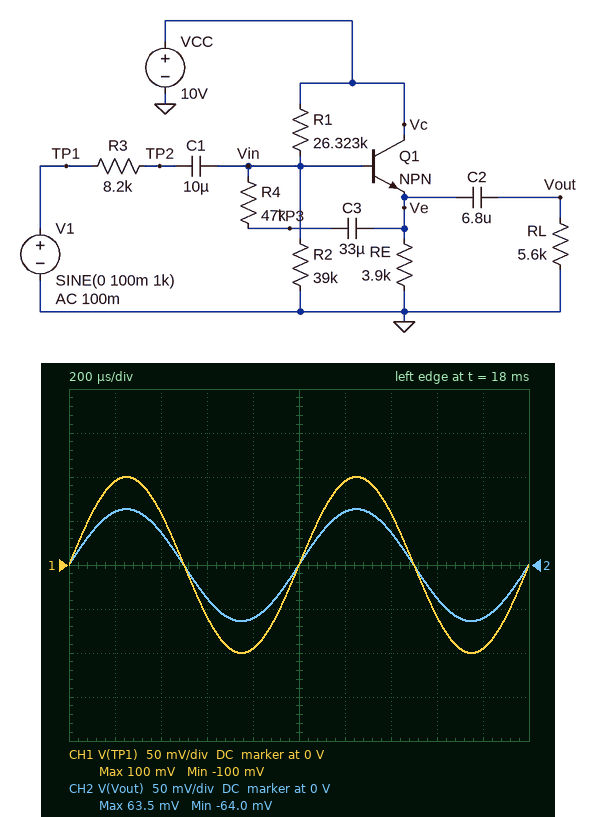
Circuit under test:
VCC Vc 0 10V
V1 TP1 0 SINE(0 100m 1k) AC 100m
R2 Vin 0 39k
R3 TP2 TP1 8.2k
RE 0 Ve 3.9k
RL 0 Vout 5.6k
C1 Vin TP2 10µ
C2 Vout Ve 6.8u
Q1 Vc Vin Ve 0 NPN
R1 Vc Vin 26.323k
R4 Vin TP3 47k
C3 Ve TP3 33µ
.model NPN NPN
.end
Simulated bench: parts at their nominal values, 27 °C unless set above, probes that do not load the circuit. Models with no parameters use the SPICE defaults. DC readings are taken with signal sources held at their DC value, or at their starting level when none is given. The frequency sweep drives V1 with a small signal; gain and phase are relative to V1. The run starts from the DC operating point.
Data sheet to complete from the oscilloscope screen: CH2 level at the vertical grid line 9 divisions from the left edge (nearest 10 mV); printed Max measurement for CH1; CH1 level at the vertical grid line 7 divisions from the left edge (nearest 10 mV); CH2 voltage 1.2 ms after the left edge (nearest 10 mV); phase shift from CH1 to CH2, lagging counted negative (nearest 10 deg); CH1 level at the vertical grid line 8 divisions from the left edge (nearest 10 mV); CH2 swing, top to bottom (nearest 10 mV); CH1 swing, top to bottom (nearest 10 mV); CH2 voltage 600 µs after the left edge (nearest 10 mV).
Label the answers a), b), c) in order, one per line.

a) -60 mV
b) 100 mV
c) 60 mV
d) 60 mV
e) 0 deg
f) -60 mV
g) 130 mV
h) 200 mV
i) -40 mV
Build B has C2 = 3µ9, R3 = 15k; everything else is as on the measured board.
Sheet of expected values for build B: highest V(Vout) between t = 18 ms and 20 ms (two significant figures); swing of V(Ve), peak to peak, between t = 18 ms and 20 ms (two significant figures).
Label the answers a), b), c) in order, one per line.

a) 49 mV
b) 98 mV
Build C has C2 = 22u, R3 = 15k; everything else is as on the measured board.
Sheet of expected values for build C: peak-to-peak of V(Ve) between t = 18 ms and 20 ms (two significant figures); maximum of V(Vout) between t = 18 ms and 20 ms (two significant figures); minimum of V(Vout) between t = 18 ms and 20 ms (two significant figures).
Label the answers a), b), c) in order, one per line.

a) 98 mV
b) 49 mV
c) -49 mV
